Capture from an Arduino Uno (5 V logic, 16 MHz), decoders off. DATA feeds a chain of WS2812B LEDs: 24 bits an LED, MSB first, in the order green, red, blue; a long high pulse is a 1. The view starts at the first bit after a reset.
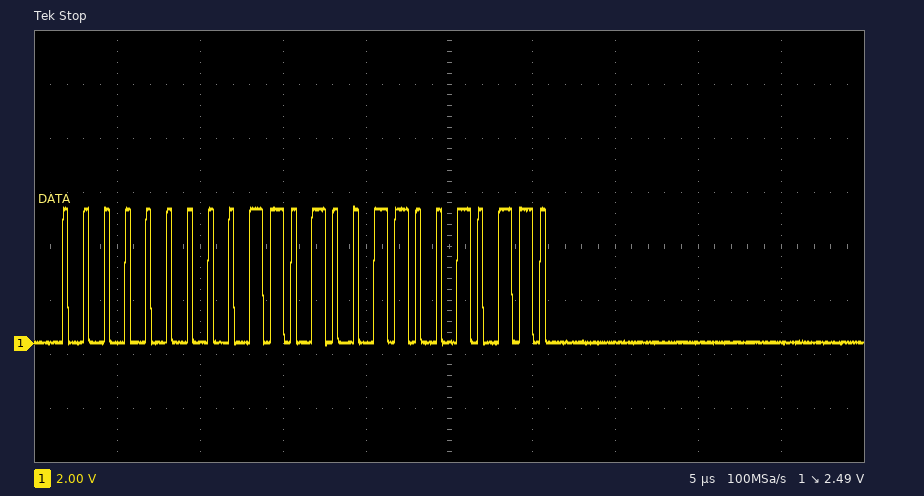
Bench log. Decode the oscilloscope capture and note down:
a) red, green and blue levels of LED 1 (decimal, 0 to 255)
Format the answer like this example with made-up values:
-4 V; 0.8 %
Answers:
105, 0, 150
